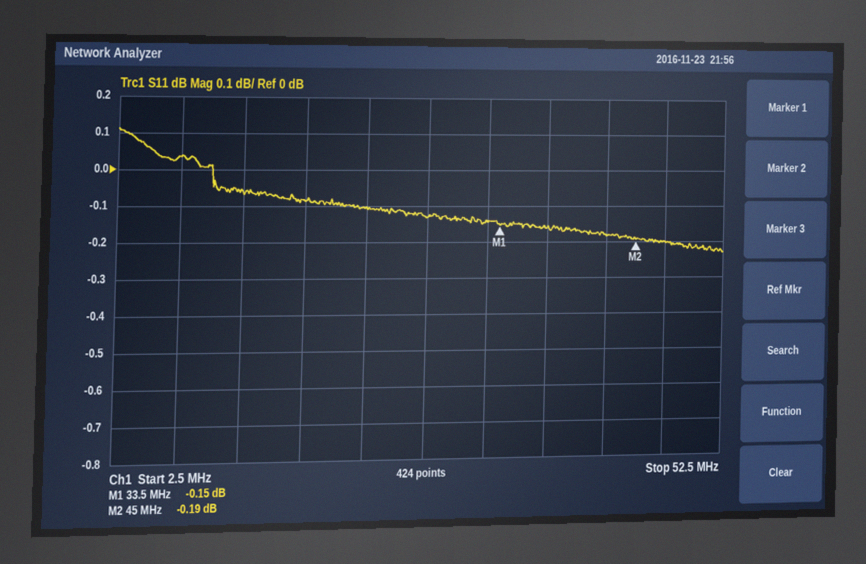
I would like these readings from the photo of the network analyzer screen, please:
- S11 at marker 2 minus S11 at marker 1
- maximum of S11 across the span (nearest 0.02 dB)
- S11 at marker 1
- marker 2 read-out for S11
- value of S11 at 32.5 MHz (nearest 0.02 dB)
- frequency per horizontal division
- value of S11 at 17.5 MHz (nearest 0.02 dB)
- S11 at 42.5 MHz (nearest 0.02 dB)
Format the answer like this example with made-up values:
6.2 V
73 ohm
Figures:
-0.04 dB
0.12 dB
-0.15 dB
-0.19 dB
-0.14 dB
5 MHz
-0.08 dB
-0.18 dB
